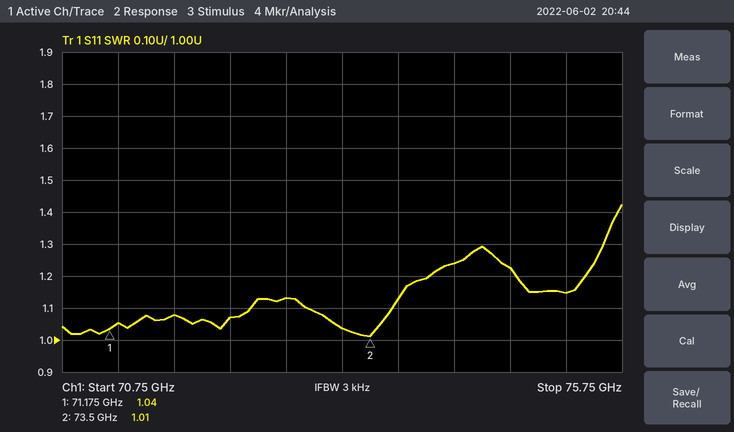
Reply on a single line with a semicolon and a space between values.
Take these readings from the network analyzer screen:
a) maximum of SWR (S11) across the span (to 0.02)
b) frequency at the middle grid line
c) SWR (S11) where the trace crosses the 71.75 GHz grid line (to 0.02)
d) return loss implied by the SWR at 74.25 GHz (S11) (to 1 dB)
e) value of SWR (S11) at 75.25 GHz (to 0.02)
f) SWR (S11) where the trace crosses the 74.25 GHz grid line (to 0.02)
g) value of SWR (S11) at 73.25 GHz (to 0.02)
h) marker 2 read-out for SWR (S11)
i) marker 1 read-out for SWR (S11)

1.42; 73.25 GHz; 1.08; 19 dB; 1.14; 1.24; 1.04; 1.01; 1.04
